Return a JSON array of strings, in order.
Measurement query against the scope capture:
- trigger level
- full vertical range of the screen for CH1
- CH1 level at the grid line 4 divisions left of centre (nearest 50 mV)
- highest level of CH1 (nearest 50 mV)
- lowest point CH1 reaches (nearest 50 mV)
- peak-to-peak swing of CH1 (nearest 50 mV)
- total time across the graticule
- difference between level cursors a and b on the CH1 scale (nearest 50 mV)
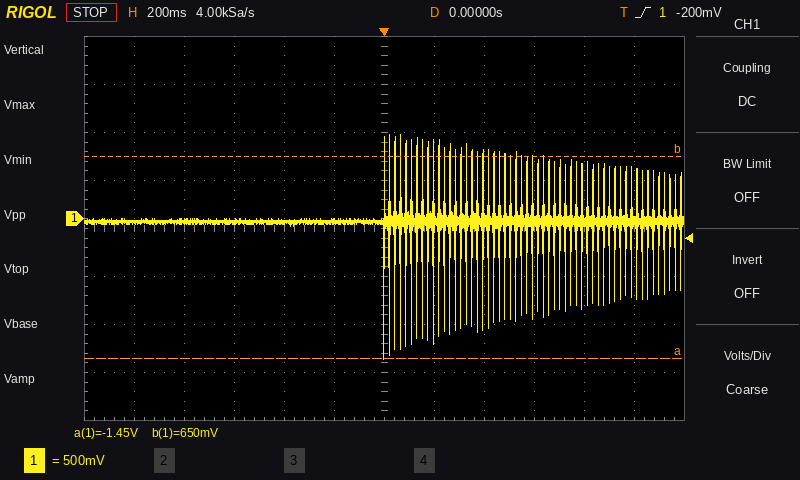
["-200 mV", "4 V", "-50 mV", "900 mV", "-1.45 V", "2.35 V", "2.4 s", "2.10 V"]
